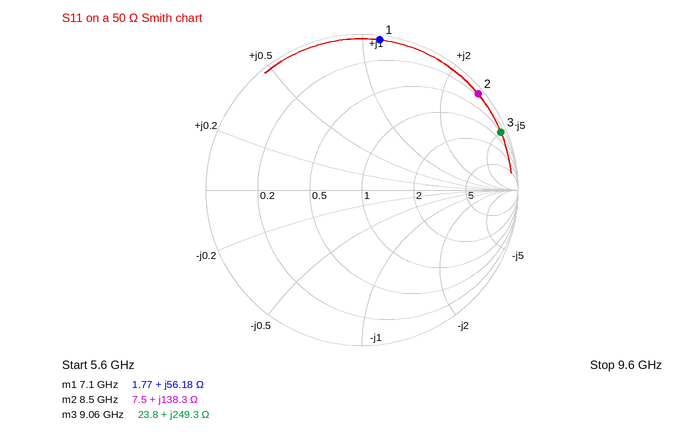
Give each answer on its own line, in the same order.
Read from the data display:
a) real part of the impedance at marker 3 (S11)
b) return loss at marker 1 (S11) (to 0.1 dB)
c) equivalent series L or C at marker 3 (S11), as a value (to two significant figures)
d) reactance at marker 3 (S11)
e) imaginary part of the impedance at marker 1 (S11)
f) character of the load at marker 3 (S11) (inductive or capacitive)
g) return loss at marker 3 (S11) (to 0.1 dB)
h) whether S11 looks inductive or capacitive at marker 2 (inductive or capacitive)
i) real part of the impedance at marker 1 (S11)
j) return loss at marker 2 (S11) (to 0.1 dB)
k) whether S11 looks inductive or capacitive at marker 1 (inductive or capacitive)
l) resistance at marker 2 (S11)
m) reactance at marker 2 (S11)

23.8 Ω
0.3 dB
4.4 nH
+249.3 Ω
+56.18 Ω
inductive
0.3 dB
inductive
1.77 Ω
0.3 dB
inductive
7.5 Ω
+138.3 Ω
